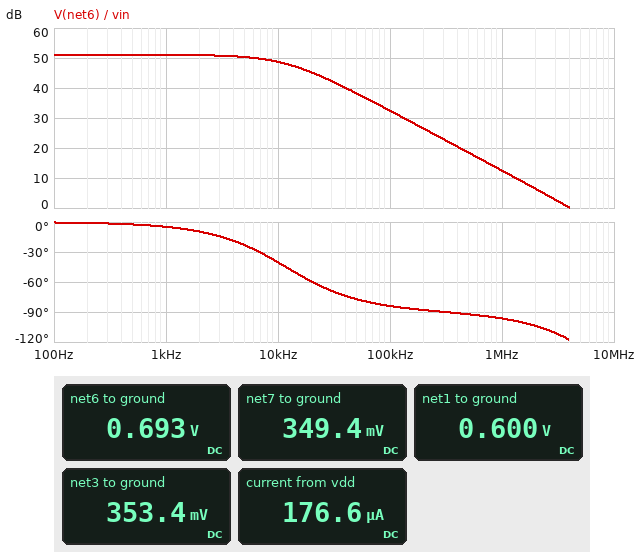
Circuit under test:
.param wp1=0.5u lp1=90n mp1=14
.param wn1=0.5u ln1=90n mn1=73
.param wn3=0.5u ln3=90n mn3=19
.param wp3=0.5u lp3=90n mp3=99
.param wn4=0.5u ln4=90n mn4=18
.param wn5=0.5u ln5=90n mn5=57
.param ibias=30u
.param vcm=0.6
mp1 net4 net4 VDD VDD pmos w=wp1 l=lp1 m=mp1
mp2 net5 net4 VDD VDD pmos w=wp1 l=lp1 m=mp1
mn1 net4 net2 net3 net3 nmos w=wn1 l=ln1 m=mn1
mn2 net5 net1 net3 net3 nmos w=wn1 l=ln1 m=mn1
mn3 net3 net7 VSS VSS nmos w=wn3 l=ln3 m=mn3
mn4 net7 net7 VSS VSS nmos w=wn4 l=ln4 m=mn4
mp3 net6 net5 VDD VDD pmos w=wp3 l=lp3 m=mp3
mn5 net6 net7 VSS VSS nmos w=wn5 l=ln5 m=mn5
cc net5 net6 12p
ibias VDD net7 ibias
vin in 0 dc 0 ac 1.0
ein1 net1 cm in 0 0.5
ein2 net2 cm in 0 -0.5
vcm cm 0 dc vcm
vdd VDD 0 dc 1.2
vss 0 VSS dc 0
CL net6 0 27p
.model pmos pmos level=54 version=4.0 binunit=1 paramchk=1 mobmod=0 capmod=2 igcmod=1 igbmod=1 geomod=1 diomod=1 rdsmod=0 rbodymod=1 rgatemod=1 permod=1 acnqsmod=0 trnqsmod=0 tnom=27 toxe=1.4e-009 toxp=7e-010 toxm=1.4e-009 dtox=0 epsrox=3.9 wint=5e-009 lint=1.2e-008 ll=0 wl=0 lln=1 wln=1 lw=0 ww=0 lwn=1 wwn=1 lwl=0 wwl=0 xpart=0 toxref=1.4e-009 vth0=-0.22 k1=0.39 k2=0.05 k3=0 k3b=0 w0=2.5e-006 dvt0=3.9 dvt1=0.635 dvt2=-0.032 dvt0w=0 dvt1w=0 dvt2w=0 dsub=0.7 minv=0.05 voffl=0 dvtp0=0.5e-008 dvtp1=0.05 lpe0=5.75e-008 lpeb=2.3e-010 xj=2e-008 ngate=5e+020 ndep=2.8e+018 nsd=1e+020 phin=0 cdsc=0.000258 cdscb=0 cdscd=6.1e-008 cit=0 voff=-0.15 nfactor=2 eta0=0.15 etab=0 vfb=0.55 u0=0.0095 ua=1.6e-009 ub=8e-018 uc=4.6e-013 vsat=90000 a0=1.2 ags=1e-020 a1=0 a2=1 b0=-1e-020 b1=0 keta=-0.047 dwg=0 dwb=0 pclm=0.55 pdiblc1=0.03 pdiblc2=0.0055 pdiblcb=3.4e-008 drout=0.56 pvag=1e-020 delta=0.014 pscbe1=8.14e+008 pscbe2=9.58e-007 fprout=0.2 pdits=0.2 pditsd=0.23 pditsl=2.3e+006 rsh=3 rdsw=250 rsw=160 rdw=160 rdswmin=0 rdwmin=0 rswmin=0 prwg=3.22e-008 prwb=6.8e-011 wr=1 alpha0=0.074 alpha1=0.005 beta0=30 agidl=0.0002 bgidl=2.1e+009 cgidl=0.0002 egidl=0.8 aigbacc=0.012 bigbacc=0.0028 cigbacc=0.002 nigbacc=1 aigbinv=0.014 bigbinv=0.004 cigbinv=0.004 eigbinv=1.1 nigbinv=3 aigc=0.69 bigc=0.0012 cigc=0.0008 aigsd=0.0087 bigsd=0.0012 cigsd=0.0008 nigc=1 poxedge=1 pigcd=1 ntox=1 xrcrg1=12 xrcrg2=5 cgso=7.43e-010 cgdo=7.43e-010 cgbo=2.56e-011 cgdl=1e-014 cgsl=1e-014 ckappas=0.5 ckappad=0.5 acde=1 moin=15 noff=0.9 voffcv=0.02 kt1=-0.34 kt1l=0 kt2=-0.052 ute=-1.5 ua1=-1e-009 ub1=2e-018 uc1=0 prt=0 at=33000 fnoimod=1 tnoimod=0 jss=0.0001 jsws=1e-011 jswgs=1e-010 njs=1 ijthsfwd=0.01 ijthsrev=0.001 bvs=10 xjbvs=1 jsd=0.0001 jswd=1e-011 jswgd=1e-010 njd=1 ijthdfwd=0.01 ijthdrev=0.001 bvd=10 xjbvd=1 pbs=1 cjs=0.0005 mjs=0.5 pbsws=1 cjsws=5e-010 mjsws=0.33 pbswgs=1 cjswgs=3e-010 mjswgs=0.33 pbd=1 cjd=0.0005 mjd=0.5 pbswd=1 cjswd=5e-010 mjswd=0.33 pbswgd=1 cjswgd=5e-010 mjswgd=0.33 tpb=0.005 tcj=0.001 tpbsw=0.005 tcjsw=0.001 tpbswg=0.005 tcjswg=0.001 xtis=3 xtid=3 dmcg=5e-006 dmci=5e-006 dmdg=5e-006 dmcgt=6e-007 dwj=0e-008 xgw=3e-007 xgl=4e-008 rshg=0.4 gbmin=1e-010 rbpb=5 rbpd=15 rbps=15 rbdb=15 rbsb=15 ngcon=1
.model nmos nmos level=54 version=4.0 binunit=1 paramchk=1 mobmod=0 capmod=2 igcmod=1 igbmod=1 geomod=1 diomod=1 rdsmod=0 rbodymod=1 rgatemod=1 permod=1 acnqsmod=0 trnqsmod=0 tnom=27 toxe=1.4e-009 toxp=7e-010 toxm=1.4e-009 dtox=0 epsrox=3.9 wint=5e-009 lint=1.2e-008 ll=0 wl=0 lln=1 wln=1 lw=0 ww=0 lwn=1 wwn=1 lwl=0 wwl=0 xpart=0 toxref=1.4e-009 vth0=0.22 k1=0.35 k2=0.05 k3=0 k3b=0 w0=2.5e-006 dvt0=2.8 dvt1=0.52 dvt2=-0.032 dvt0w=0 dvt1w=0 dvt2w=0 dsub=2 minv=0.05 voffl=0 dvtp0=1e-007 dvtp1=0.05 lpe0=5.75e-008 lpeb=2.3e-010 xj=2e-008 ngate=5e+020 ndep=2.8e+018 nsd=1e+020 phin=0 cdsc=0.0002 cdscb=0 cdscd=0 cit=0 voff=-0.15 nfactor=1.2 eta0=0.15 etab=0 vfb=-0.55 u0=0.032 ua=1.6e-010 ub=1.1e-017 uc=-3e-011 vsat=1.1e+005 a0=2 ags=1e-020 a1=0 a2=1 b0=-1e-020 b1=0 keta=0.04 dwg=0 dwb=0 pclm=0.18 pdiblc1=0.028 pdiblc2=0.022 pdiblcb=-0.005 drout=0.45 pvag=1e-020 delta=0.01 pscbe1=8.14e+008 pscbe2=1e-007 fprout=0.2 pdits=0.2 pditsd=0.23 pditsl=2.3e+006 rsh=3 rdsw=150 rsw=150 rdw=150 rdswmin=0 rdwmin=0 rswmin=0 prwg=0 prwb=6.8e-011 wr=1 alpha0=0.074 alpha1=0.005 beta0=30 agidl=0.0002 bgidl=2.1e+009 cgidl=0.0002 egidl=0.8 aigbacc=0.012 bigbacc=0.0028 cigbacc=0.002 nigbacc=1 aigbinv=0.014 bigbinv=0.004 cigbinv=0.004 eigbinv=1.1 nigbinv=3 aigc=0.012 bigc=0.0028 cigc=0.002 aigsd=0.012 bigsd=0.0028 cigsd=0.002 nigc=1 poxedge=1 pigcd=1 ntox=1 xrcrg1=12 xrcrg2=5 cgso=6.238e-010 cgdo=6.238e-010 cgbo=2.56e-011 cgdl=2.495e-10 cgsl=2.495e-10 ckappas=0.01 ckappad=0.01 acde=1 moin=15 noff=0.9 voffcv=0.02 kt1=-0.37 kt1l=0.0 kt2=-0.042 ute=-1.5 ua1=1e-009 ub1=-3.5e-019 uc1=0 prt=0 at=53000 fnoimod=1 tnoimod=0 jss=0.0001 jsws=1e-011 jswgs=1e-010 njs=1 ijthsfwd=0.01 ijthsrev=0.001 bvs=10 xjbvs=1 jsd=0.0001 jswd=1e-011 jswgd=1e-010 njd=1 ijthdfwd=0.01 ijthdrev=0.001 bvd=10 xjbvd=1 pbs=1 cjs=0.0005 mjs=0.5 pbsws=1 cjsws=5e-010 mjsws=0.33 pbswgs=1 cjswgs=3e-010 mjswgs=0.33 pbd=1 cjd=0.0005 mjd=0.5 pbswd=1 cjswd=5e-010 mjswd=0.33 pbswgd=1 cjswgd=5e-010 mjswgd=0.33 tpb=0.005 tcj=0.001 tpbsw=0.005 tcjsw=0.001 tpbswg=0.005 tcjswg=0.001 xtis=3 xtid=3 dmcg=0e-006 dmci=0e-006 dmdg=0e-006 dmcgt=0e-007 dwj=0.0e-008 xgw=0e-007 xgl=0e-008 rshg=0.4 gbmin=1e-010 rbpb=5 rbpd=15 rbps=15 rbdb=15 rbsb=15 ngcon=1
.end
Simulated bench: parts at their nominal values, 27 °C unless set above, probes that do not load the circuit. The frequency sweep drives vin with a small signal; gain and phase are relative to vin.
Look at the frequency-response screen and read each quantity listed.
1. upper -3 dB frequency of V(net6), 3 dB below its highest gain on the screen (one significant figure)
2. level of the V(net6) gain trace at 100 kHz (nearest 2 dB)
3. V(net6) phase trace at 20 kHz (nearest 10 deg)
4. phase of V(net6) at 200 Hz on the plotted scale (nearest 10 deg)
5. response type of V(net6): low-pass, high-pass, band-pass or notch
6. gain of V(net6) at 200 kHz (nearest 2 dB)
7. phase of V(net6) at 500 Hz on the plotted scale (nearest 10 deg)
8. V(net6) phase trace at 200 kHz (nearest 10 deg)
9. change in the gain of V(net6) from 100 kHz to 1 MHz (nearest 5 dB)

10 kHz
32 dB
-60 deg
0 deg
low-pass
26 dB
0 deg
-90 deg
-20 dB
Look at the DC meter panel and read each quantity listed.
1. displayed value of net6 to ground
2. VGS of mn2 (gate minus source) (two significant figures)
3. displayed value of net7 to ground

0.693 V
250 mV
349.4 mV
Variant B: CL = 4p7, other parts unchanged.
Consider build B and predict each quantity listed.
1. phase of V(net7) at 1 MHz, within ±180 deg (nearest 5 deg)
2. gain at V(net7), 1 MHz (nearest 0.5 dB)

-85 deg
-42.0 dB
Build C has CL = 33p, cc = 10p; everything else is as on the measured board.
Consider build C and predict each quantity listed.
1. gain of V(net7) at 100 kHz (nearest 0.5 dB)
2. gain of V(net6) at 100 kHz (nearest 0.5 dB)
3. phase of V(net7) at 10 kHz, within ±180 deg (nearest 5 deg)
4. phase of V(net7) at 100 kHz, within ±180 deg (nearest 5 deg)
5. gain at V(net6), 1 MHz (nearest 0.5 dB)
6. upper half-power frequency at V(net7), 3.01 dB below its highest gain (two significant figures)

-21.0 dB
34.0 dB
-35 deg
-80 deg
14.0 dB
14 kHz
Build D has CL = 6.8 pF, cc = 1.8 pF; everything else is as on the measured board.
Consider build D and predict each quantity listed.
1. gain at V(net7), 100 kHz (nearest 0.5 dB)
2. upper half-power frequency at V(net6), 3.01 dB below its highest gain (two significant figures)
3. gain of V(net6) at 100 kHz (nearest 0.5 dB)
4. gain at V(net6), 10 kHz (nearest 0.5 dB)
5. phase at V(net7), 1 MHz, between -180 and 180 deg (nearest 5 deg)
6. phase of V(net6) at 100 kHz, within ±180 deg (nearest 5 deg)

-8.0 dB
76 kHz
46.5 dB
51.0 dB
-80 deg
-55 deg
